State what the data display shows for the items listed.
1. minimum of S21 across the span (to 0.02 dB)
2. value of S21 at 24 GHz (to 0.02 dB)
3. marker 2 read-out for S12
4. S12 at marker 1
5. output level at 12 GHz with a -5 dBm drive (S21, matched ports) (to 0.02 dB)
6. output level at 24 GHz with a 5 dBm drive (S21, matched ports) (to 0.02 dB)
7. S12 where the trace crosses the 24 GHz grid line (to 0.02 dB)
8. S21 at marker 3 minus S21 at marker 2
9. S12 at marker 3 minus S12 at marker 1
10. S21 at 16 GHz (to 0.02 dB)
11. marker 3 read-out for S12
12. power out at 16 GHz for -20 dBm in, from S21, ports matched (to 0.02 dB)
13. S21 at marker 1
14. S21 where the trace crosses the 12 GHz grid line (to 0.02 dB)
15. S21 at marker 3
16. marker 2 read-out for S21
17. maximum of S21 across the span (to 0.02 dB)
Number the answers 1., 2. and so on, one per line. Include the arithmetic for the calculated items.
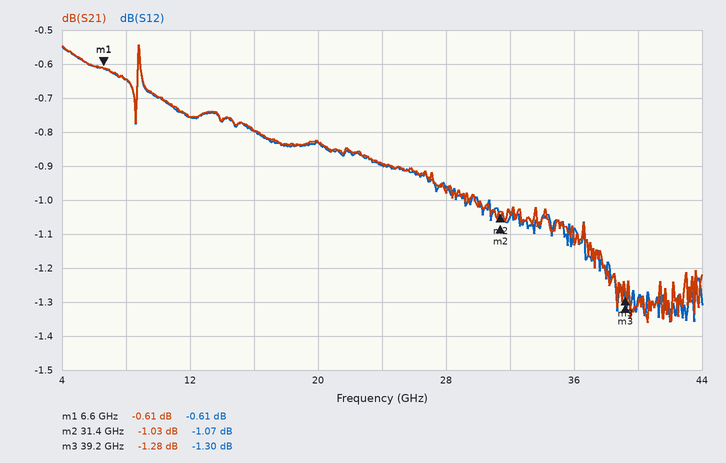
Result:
1. -1.36 dB
2. -0.90 dB
3. -1.07 dB
4. -0.61 dB
5. -5 dBm + (-0.76 dB) = -5.76 dBm
6. 5 dBm + (-0.90 dB) = 4.10 dBm
7. -0.90 dB
8. -1.28 − (-1.03) = -0.25 dB
9. -1.3 − (-0.61) = -0.69 dB
10. -0.80 dB
11. -1.30 dB
12. -20 dBm + (-0.80 dB) = -20.80 dBm
13. -0.61 dB
14. -0.76 dB
15. -1.28 dB
16. -1.03 dB
17. -0.54 dB
